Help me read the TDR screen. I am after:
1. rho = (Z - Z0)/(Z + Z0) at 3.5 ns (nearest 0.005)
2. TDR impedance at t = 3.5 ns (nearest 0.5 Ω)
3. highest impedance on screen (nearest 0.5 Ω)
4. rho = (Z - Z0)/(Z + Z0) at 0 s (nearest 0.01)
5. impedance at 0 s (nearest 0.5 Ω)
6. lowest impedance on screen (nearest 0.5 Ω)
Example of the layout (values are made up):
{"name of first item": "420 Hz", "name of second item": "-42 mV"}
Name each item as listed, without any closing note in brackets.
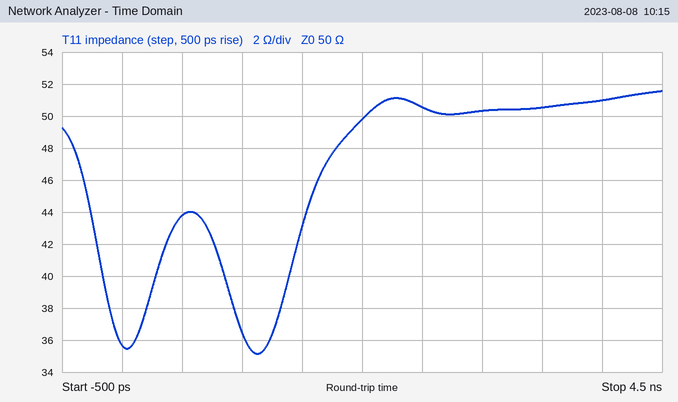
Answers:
{"rho = (Z - Z0)/(Z + Z0) at 3.5 ns": "+0.005", "TDR impedance at t = 3.5 ns": "50.5 Ω", "highest impedance on screen": "51.5 Ω", "rho = (Z - Z0)/(Z + Z0) at 0 s": "-0.17", "impedance at 0 s": "35.5 Ω", "lowest impedance on screen": "35.0 Ω"}
